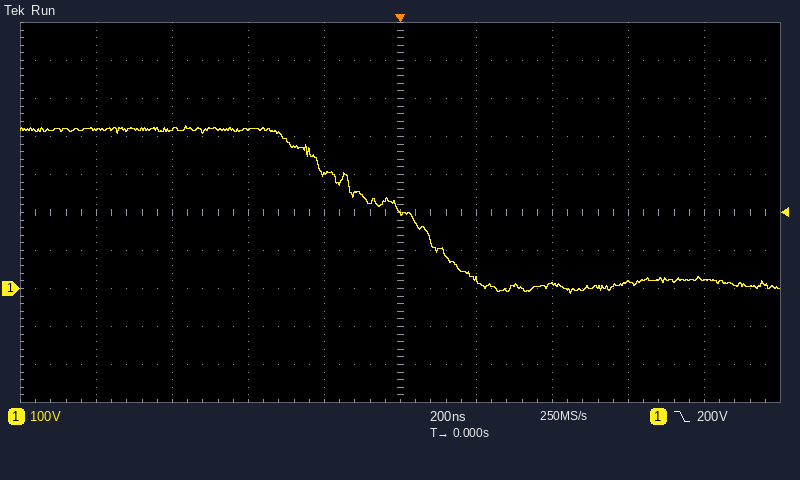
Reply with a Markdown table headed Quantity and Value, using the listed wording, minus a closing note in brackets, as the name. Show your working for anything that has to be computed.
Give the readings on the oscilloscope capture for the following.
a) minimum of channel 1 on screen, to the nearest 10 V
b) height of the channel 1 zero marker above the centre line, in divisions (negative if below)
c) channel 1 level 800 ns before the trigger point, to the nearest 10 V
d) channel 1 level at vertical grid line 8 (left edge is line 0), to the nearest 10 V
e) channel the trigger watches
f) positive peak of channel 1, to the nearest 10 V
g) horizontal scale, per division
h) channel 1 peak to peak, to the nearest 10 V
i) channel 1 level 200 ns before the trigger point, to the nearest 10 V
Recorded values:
| Quantity | Value |
|---|---|
| minimum of channel 1 on screen, to the nearest 10 V | -10 V |
| height of the channel 1 zero marker above the centre line, in divisions | -2.0 div |
| channel 1 level 800 ns before the trigger point, to the nearest 10 V | 420 V |
| channel 1 level at vertical grid line 8 (left edge is line 0), to the nearest 10 V | 20 V |
| channel the trigger watches | channel 1 |
| positive peak of channel 1, to the nearest 10 V | 430 V |
| horizontal scale, per division | 200 ns |
| channel 1 peak to peak, to the nearest 10 V | 430 V − (-10 V) = 440 V |
| channel 1 level 200 ns before the trigger point, to the nearest 10 V | 300 V |
